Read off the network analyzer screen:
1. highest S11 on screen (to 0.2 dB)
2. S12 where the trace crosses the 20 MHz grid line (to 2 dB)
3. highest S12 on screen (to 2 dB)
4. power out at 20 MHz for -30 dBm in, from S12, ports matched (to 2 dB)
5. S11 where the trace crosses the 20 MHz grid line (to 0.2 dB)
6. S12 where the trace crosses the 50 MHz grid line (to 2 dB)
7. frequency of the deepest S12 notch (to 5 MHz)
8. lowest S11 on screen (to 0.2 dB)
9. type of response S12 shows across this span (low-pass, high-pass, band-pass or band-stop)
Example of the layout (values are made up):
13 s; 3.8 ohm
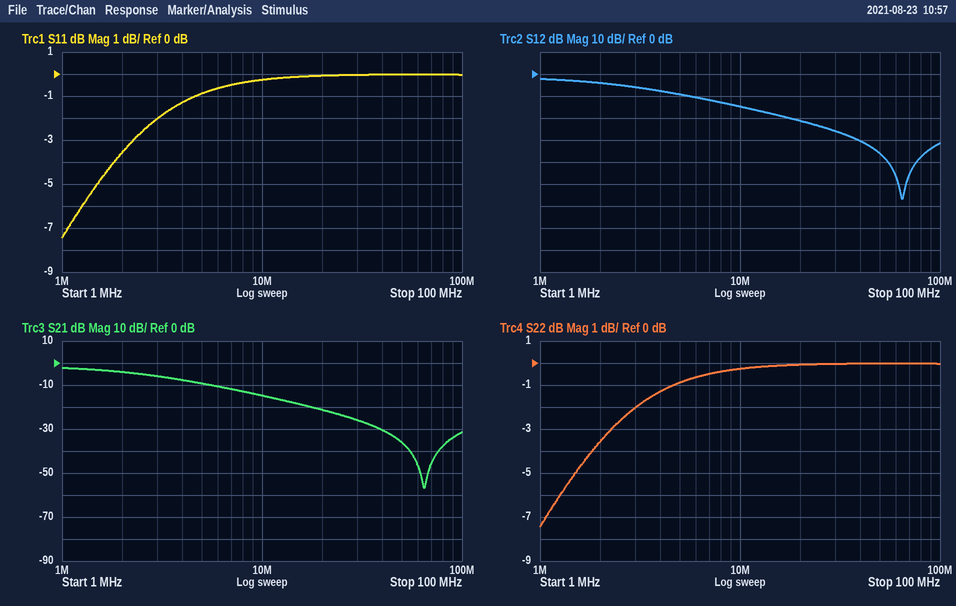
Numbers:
0.0 dB; -22 dB; -2 dB; -52 dBm; 0.0 dB; -36 dB; 65 MHz; -7.4 dB; low-pass
